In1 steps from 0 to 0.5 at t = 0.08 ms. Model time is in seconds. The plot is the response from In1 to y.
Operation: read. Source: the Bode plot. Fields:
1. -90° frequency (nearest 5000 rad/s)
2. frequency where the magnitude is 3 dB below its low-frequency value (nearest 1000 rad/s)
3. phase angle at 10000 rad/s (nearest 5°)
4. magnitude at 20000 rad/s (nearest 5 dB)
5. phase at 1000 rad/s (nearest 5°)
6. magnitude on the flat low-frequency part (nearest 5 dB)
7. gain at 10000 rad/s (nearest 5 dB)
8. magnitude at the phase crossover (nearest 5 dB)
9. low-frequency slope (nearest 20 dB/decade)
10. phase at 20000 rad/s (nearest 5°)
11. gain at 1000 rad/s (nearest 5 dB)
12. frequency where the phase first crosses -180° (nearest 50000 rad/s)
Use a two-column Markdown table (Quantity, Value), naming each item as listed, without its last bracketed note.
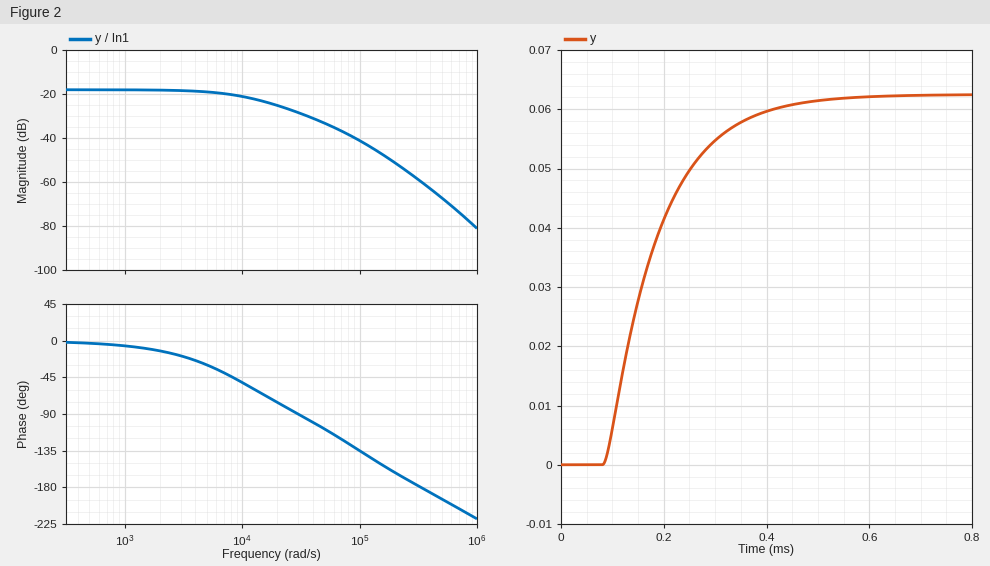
| Quantity | Value |
|---|---|
| -90° frequency | 30000 rad/s |
| frequency where the magnitude is 3 dB below its low-frequency value | 10000 rad/s |
| phase angle at 10000 rad/s | -50° |
| magnitude at 20000 rad/s | -25 dB |
| phase at 1000 rad/s | -5° |
| magnitude on the flat low-frequency part | -20 dB |
| gain at 10000 rad/s | -20 dB |
| magnitude at the phase crossover | -60 dB |
| low-frequency slope | 0 dB/decade |
| phase at 20000 rad/s | -75° |
| gain at 1000 rad/s | -20 dB |
| frequency where the phase first crosses -180° | 350000 rad/s |
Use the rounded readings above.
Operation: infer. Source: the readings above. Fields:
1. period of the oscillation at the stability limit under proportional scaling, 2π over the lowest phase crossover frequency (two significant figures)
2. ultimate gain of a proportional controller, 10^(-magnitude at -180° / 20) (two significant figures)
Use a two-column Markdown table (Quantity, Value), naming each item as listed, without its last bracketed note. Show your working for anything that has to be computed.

| Quantity | Value |
|---|---|
| period of the oscillation at the stability limit under proportional scaling, 2π over the lowest phase crossover frequency | 2π / 350000 = 0.000018 s |
| ultimate gain of a proportional controller, 10^(-magnitude at -180° / 20) | 10^(60 / 20) = 1000 |
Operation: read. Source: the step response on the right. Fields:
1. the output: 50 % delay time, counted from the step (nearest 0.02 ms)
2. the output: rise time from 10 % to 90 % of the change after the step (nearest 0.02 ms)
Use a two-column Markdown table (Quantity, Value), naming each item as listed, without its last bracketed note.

| Quantity | Value |
|---|---|
| the output: 50 % delay time, counted from the step | 0.08 ms |
| the output: rise time from 10 % to 90 % of the change after the step | 0.22 ms |
